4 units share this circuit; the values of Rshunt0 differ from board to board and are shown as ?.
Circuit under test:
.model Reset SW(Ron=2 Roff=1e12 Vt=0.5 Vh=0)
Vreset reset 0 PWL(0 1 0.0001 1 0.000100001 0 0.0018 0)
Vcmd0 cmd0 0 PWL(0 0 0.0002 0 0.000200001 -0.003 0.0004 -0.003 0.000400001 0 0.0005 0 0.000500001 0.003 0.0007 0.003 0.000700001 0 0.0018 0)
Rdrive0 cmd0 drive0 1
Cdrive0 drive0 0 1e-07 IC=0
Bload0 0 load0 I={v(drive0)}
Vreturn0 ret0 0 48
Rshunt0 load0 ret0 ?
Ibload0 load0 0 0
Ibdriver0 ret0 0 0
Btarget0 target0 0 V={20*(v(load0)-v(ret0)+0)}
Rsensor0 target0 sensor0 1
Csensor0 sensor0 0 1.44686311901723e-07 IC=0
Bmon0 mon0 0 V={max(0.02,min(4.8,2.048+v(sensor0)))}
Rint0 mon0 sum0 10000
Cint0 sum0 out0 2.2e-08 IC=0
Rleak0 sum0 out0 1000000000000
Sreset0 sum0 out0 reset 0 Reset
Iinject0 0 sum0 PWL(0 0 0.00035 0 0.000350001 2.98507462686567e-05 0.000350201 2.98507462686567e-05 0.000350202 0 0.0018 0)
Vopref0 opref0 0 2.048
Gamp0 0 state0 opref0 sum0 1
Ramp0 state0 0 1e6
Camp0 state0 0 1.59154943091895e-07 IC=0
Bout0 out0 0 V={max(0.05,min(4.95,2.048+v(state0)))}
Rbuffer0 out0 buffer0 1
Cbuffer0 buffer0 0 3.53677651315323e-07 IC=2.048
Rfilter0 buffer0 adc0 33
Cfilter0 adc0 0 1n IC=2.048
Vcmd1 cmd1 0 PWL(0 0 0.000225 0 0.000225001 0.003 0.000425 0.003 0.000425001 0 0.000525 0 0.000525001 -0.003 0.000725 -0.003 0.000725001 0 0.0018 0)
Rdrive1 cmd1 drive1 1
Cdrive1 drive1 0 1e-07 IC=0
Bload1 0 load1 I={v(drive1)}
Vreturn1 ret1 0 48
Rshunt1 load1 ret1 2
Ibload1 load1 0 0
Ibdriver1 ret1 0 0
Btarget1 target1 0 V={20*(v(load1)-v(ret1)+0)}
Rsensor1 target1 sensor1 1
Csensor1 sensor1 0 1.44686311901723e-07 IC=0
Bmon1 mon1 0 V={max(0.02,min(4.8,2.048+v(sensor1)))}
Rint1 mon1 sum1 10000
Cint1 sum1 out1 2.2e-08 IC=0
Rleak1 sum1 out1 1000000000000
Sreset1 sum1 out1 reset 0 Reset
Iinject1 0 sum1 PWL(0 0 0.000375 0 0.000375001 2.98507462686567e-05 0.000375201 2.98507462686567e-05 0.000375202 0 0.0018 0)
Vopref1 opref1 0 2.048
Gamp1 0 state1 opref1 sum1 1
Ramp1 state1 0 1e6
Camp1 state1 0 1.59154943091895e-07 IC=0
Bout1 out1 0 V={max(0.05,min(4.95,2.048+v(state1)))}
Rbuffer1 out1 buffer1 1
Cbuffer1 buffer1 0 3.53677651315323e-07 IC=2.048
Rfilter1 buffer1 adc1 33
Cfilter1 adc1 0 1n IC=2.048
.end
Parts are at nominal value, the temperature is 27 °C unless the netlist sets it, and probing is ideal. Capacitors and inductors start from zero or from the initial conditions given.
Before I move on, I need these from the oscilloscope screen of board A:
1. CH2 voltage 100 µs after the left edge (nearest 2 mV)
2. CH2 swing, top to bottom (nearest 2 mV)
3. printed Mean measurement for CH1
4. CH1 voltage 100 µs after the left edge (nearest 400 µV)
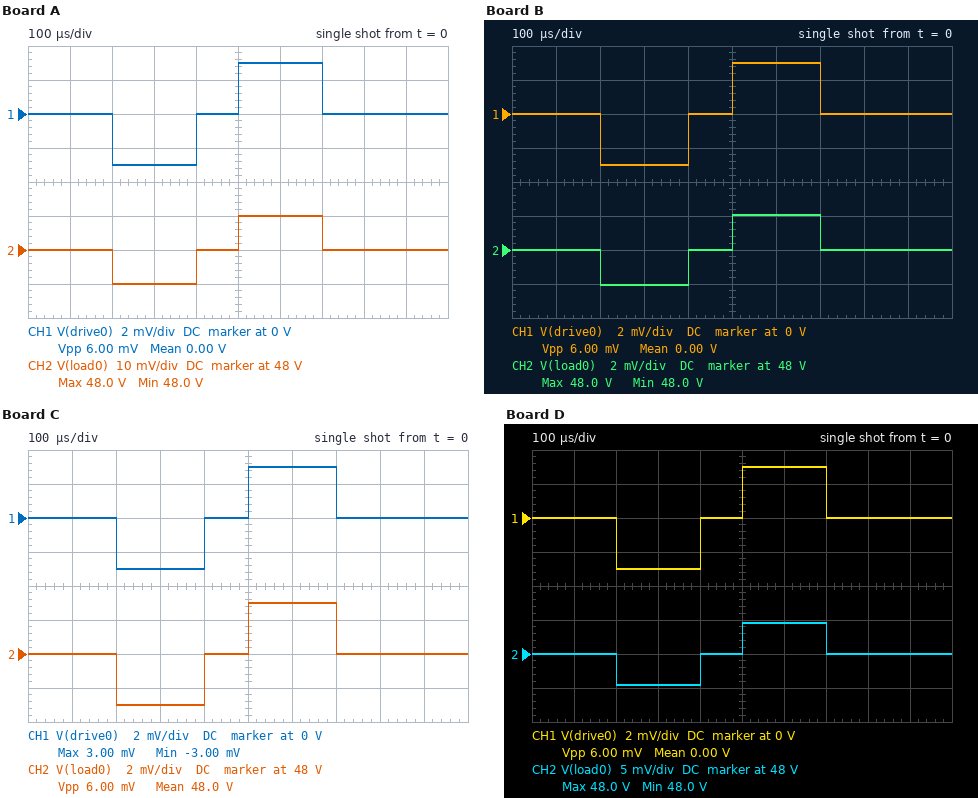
48.000 V
20 mV
0.00 V
0 V
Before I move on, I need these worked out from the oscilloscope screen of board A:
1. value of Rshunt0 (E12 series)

3.3 Ω
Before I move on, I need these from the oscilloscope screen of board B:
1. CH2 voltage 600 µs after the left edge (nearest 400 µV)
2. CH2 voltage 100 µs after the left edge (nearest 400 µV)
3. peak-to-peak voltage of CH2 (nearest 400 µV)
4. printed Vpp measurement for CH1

48.0020 V
48.0000 V
4.0 mV
6.00 mV
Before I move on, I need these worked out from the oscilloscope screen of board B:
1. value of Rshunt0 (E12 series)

0.68 Ω
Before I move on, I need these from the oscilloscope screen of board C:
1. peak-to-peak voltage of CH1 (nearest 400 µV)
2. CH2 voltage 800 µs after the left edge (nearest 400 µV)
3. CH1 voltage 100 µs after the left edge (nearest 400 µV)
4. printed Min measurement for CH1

6.0 mV
48.0000 V
0 V
-3.00 mV
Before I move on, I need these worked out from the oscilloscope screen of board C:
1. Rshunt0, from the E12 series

1 Ω
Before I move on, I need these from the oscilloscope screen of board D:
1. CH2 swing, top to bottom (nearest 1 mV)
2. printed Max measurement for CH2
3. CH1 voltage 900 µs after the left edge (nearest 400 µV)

9 mV
48.0 V
0 V
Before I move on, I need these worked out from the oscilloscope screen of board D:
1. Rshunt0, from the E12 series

1.5 Ω
